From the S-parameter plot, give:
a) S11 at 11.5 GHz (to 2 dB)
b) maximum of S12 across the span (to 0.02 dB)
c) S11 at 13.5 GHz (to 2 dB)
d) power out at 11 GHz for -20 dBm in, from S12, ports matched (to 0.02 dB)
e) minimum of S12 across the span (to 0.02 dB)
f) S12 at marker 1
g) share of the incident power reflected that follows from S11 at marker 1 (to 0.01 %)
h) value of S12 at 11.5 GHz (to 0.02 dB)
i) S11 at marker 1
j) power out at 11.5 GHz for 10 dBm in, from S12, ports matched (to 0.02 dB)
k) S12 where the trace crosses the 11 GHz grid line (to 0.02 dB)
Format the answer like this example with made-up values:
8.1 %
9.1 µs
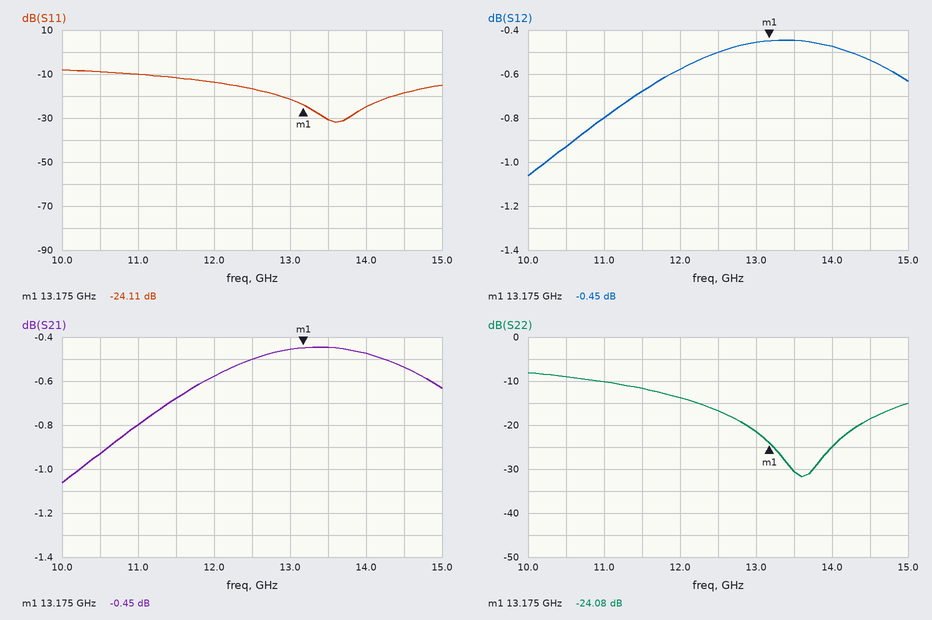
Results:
-12 dB
-0.44 dB
-30 dB
-20.80 dBm
-1.06 dB
-0.45 dB
0.39 %
-0.68 dB
-24.11 dB
9.32 dBm
-0.80 dB
